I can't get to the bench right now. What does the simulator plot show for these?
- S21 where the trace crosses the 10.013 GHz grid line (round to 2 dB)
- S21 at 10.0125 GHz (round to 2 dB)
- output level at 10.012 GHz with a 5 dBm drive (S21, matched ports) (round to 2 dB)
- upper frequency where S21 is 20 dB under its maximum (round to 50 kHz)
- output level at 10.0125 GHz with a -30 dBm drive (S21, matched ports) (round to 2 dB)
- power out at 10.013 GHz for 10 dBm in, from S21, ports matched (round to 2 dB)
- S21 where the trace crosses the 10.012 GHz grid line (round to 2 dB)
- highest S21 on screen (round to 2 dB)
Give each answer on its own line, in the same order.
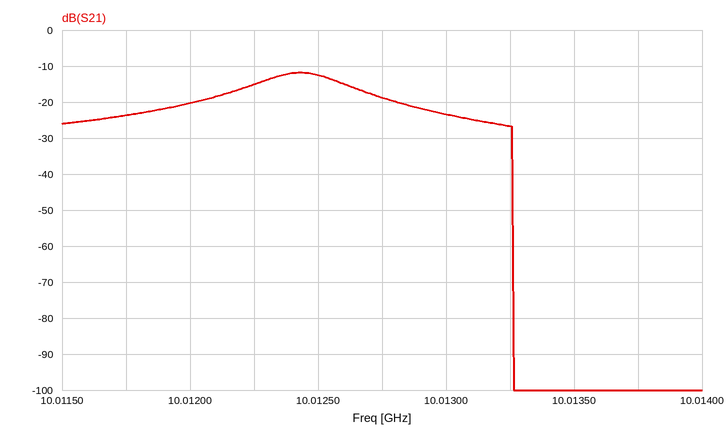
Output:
-24 dB
-12 dB
-16 dBm
10.01325 GHz
-42 dBm
-14 dBm
-20 dB
-12 dB
